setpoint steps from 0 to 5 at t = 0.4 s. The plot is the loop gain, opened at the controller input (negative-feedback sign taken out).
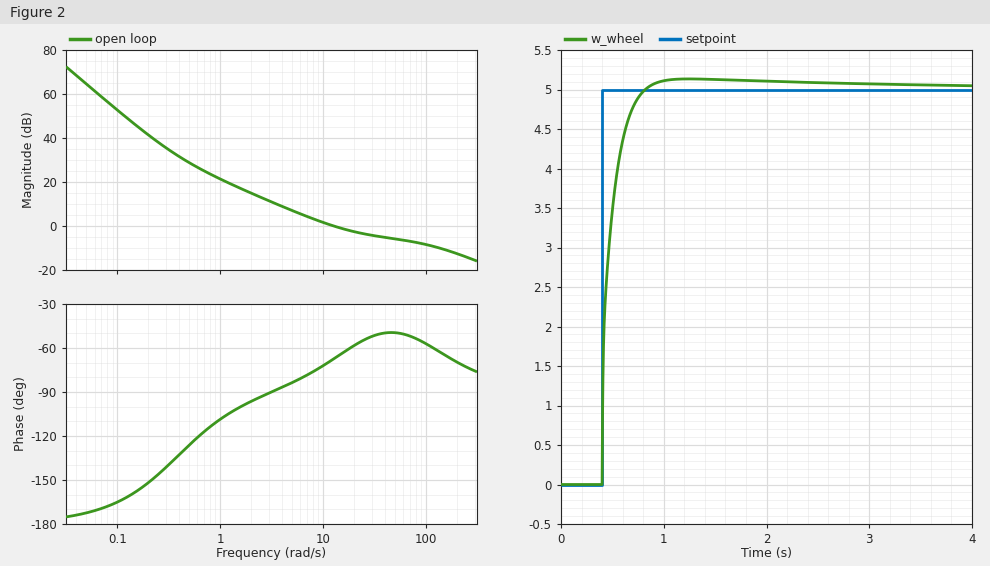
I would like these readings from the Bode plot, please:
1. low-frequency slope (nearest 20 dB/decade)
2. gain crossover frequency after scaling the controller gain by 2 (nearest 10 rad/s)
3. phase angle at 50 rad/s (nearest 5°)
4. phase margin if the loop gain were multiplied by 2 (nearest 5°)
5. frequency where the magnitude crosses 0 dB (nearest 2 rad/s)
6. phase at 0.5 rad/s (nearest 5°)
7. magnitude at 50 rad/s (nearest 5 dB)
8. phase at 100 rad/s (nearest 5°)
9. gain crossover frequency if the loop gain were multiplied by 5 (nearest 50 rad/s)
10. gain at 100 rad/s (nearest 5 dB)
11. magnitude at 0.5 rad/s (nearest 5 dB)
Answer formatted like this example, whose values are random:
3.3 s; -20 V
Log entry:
-40 dB/decade; 50 rad/s; -50°; 130°; 12 rad/s; -125°; -5 dB; -55°; 250 rad/s; -10 dB; 30 dB
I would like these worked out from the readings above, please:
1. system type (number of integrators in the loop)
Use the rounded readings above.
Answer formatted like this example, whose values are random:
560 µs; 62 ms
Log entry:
2
